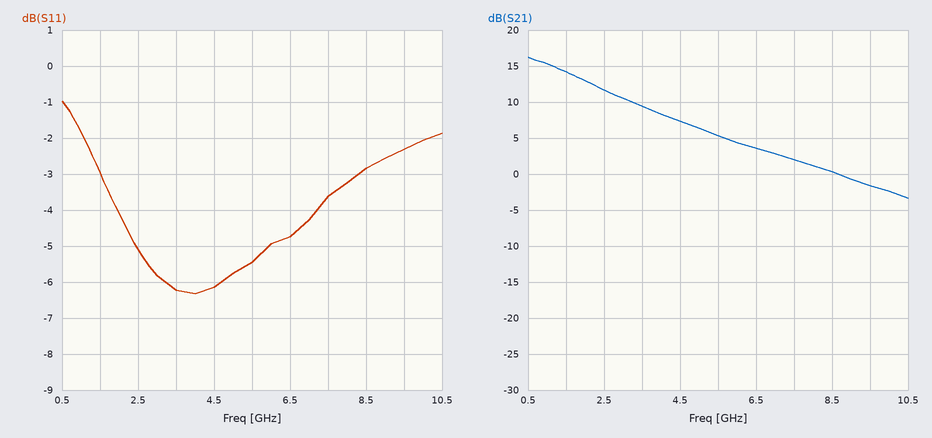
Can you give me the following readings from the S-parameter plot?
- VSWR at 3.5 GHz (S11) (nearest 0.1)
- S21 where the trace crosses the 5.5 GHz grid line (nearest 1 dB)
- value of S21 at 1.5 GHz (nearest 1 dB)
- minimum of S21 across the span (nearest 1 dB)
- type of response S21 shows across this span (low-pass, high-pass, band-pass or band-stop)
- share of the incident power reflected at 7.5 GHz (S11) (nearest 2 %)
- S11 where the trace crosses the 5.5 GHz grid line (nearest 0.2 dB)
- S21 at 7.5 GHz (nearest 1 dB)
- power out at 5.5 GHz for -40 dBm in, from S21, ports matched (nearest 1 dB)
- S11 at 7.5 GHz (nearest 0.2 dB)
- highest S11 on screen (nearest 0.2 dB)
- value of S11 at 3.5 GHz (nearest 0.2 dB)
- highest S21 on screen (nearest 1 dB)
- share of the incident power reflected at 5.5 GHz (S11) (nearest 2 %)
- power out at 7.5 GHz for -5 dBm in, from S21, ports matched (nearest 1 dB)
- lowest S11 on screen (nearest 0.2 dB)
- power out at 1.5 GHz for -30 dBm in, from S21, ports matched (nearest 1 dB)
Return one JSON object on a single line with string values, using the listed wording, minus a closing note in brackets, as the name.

{"VSWR at 3.5 GHz (S11)": "2.9", "S21 where the trace crosses the 5.5 GHz grid line": "5 dB", "value of S21 at 1.5 GHz": "14 dB", "minimum of S21 across the span": "-3 dB", "type of response S21 shows across this span": "low-pass", "share of the incident power reflected at 7.5 GHz (S11)": "44 %", "S11 where the trace crosses the 5.5 GHz grid line": "-5.4 dB", "S21 at 7.5 GHz": "2 dB", "power out at 5.5 GHz for -40 dBm in, from S21, ports matched": "-35 dBm", "S11 at 7.5 GHz": "-3.6 dB", "highest S11 on screen": "-1.0 dB", "value of S11 at 3.5 GHz": "-6.2 dB", "highest S21 on screen": "16 dB", "share of the incident power reflected at 5.5 GHz (S11)": "28 %", "power out at 7.5 GHz for -5 dBm in, from S21, ports matched": "-3 dBm", "lowest S11 on screen": "-6.4 dB", "power out at 1.5 GHz for -30 dBm in, from S21, ports matched": "-16 dBm"}
